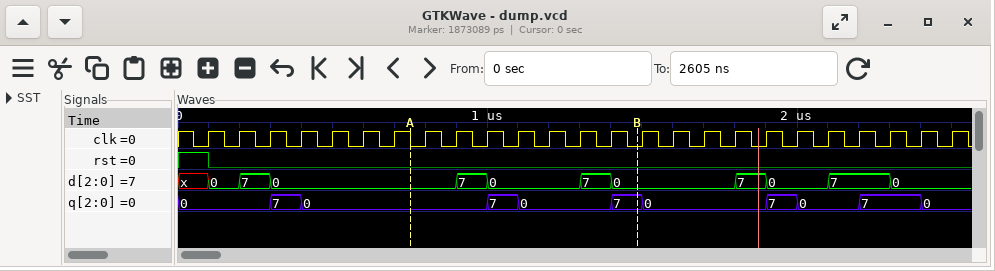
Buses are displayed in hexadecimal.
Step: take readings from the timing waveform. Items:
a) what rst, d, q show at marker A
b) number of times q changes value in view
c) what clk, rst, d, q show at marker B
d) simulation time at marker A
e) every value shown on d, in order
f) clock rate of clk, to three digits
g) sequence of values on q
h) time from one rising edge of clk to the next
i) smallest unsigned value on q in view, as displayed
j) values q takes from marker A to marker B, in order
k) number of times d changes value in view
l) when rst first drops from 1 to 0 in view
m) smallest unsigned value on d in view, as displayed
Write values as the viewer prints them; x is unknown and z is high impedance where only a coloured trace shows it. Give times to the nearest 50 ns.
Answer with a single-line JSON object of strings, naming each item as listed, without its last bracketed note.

{"what rst, d, q show at marker A": "rst=0, d=0, q=0", "number of times q changes value in view": "10", "what clk, rst, d, q show at marker B": "clk=0, rst=0, d=0, q=7", "simulation time at marker A": "750 ns", "every value shown on d, in order": "x, 0, 7, 0, 7, 0, 7, 0, 7, 0, 7, 0", "clock rate of clk, to three digits": "10.0 MHz", "sequence of values on q": "0, 7, 0, 7, 0, 7, 0, 7, 0, 7, 0", "time from one rising edge of clk to the next": "100 ns", "smallest unsigned value on q in view, as displayed": "0", "values q takes from marker A to marker B, in order": "0, 7, 0, 7", "number of times d changes value in view": "11", "when rst first drops from 1 to 0 in view": "100 ns", "smallest unsigned value on d in view, as displayed": "0"}
